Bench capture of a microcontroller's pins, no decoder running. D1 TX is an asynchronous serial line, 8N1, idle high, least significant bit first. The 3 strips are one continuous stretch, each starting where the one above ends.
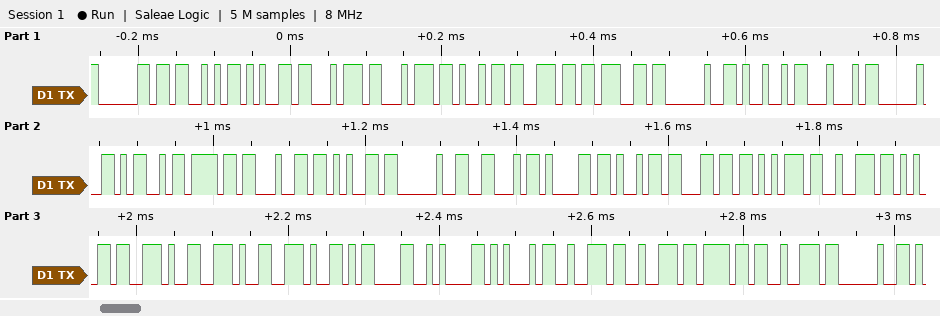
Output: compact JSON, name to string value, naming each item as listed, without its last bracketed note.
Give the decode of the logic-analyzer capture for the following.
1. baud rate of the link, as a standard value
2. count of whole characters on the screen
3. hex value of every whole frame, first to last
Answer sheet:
{"baud rate of the link, as a standard value": "115200 baud", "count of whole characters on the screen": "35", "hex value of every whole frame, first to last": "60 53 65 74 74 69 6E 67 20 49 44 20 4D 6F 64 65 20 46 61 69 6C 75 72 65 2E 2E 2E 0D 0A 45 72 72 6F 72 20"}
